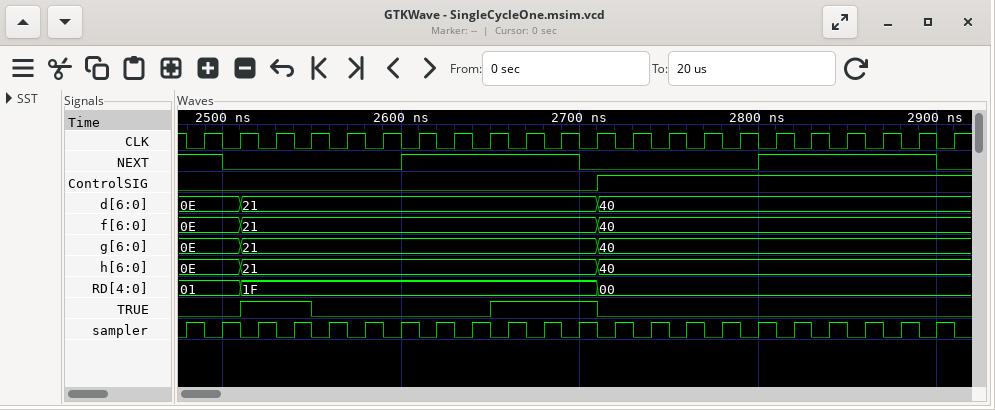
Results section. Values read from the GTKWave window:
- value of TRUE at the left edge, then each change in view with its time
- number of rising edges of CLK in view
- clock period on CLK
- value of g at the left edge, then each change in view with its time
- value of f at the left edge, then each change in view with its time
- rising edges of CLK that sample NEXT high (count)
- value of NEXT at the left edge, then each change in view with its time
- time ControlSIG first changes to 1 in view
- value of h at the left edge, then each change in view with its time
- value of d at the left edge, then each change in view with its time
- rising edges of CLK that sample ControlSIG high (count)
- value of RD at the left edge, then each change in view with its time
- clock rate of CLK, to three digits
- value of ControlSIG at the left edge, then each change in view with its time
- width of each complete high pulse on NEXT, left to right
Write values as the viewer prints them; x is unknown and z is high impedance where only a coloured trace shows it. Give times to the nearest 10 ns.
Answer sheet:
0, 1 at 2510 ns, 0 at 2550 ns, 1 at 2650 ns, 0 at 2710 ns
22
20 ns
0E, 21 at 2510 ns, 40 at 2710 ns
0E, 21 at 2510 ns, 40 at 2710 ns
11
1, 0 at 2500 ns, 1 at 2600 ns, 0 at 2700 ns, 1 at 2800 ns, 0 at 2900 ns
2710 ns
0E, 21 at 2510 ns, 40 at 2710 ns
0E, 21 at 2510 ns, 40 at 2710 ns
10
01, 1F at 2510 ns, 00 at 2710 ns
50.0 MHz
0, 1 at 2710 ns
100 ns, 100 ns
